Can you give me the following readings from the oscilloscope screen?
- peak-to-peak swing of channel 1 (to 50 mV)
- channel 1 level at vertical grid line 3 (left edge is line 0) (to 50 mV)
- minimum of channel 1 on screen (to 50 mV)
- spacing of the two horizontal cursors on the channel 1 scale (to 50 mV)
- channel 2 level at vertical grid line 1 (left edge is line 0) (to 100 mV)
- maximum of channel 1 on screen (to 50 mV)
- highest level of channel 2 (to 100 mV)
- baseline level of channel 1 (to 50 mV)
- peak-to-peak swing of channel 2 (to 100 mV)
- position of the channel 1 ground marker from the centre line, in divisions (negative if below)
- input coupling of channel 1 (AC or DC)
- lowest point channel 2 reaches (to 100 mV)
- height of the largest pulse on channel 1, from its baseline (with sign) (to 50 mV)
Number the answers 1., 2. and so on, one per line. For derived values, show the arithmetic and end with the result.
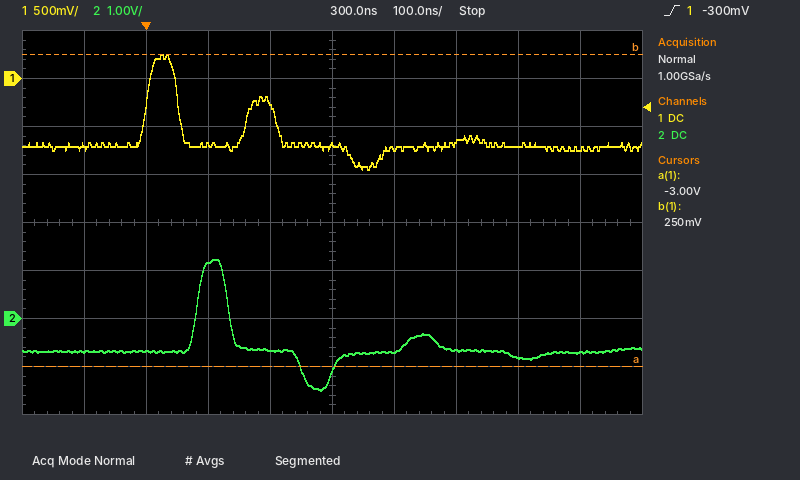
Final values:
1. 250 mV − (-950 mV) = 1.20 V
2. -700 mV
3. -950 mV
4. 3.25 V
5. -700 mV
6. 250 mV
7. 1.2 V
8. -700 mV
9. 1.2 V − (-1.5 V) = 2.7 V
10. +3.0 div
11. DC
12. -1.5 V
13. 250 mV − (-700 mV) = +950 mV
